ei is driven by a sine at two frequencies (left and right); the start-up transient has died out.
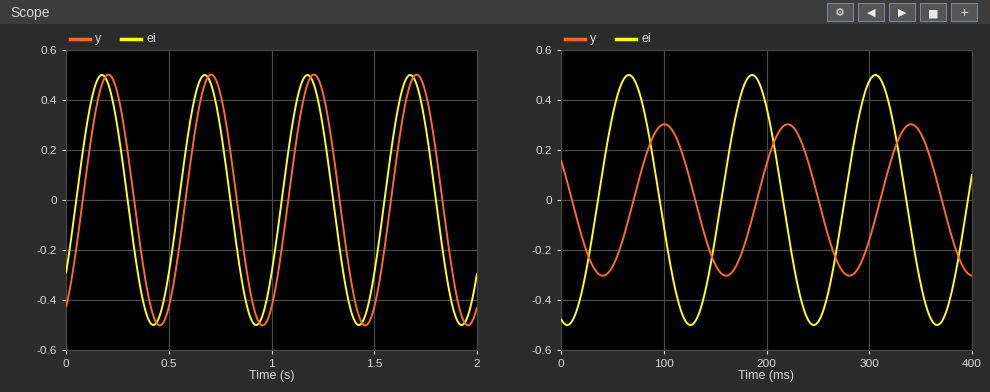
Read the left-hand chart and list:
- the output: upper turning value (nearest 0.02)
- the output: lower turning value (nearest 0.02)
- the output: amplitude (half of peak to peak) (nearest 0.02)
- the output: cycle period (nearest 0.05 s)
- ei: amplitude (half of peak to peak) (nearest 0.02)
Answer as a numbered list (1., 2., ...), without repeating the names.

1. 0.50
2. -0.50
3. 0.50
4. 0.50 s
5. 0.50
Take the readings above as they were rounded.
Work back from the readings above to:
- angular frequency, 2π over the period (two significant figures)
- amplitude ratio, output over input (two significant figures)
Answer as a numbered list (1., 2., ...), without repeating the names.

1. 13 rad/s
2. 1.0
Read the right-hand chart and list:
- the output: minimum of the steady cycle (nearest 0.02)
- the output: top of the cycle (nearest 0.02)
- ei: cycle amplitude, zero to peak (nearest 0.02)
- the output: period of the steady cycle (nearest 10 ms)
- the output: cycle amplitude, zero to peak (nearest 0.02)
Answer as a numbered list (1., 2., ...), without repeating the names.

1. -0.30
2. 0.30
3. 0.50
4. 120 ms
5. 0.30
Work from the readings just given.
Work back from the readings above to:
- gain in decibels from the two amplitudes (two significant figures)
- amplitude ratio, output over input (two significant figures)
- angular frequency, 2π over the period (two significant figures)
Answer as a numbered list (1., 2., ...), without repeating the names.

1. -4.4 dB
2. 0.60
3. 0.052 rad/ms
